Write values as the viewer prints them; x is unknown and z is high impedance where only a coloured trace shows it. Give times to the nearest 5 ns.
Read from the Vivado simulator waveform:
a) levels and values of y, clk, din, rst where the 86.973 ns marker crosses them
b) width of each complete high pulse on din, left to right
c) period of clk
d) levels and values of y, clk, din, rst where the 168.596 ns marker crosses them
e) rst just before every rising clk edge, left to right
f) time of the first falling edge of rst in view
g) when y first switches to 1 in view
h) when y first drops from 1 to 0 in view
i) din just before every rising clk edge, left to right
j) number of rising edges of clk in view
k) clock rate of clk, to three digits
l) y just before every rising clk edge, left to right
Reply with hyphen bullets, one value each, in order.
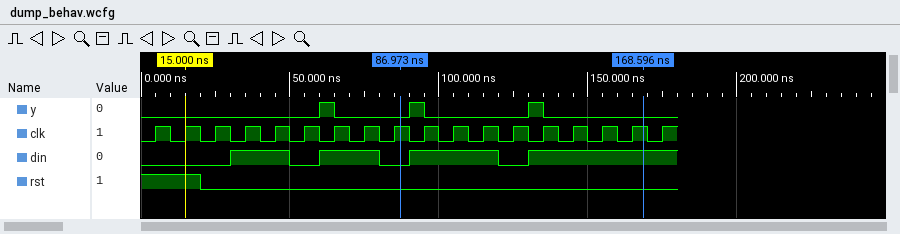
- y=0, clk=1, din=0, rst=0
- 20 ns, 20 ns, 30 ns
- 10 ns
- y=0, clk=1, din=1, rst=0
- 1 1 0 0 0 0 0 0 0 0 0 0 0 0 0 0 0 0
- 20 ns
- 60 ns
- 65 ns
- 0 0 0 1 1 0 1 1 0 1 1 1 0 1 1 1 1 1
- 18
- 100 MHz
- 0 0 0 0 0 0 1 0 0 1 0 0 0 1 0 0 0 0
